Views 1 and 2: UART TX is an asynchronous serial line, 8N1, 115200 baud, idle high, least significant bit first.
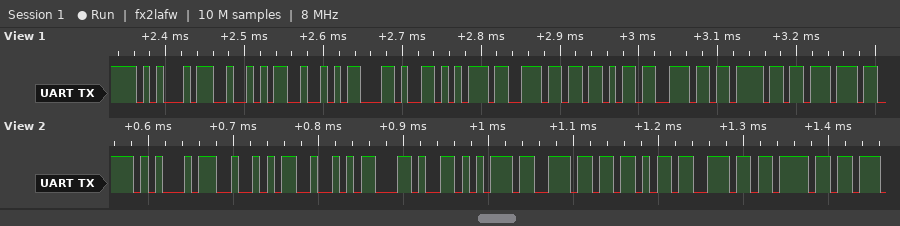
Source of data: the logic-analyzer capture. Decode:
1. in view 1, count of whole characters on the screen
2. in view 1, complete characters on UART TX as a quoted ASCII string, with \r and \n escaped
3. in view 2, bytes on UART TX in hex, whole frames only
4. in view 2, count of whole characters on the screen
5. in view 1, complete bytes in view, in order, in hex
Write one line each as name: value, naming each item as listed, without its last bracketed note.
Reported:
in view 1, count of whole characters on the screen: 10
in view 1, complete characters on UART TX as a quoted ASCII string, with \r and \n escaped: "ERR,unknow"
in view 2, bytes on UART TX in hex, whole frames only: 45 52 52 2C 75 6E 6B 6E 6F
in view 2, count of whole characters on the screen: 9
in view 1, complete bytes in view, in order, in hex: 0x45 0x52 0x52 0x2C 0x75 0x6E 0x6B 0x6E 0x6F 0x77
